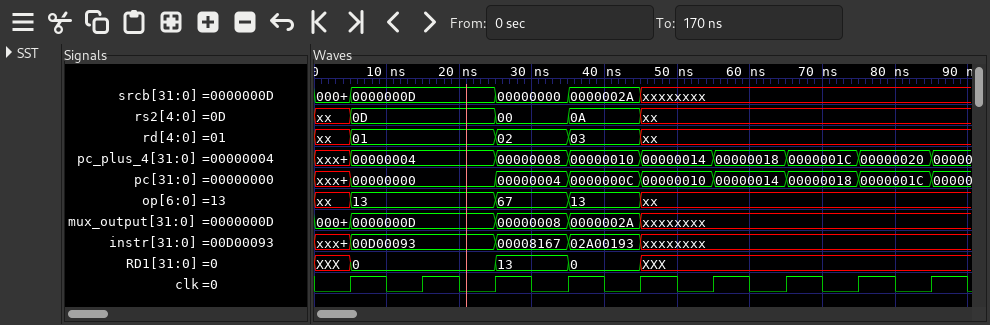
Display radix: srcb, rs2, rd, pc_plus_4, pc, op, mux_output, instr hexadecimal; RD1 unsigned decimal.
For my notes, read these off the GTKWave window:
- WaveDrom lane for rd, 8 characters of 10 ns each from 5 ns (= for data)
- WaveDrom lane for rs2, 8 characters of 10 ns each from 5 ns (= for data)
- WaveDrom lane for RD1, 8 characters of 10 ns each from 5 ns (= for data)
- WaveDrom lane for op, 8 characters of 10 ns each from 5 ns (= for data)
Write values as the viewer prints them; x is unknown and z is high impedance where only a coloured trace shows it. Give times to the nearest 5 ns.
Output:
{name: 'rd', wave: '=.==x...', data: '01 02 03'}
{name: 'rs2', wave: '=.==x...', data: '0D 00 0A'}
{name: 'RD1', wave: '=.==x...', data: '0 13 0'}
{name: 'op', wave: '=.==x...', data: '13 67 13'}
